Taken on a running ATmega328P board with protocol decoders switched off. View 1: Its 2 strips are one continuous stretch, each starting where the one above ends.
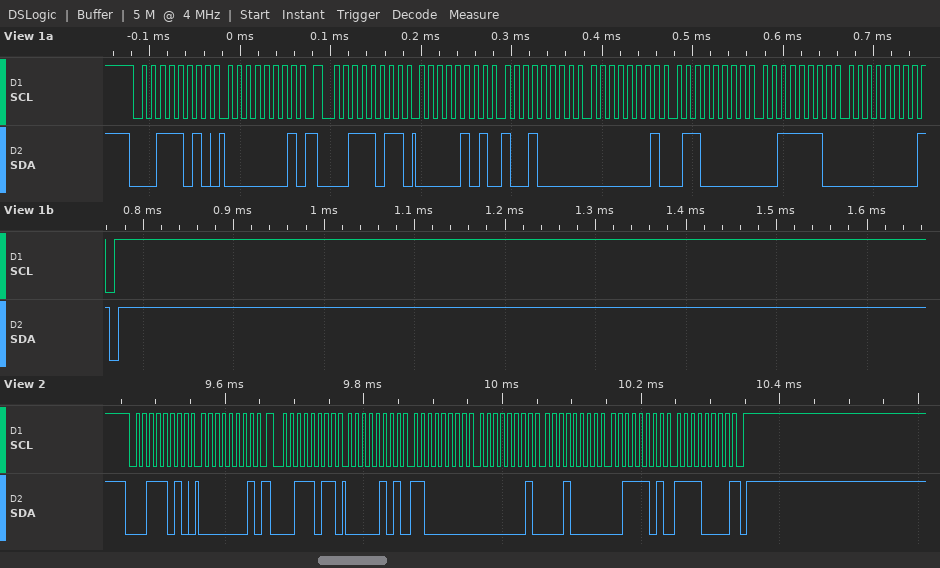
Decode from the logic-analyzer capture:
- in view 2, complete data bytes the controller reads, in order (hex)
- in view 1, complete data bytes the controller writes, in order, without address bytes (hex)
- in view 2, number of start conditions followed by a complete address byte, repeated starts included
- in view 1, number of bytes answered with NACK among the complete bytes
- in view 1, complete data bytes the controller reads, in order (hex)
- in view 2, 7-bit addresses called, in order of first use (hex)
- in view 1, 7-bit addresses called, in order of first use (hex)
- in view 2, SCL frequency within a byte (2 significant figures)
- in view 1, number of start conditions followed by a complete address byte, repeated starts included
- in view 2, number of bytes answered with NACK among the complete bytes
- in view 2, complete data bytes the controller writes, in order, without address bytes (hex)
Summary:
05 C0 01 10 3D F0
01
2
1
05 90 01 60 3E 00
0x1D
0x1D
100 kHz
2
1
01
